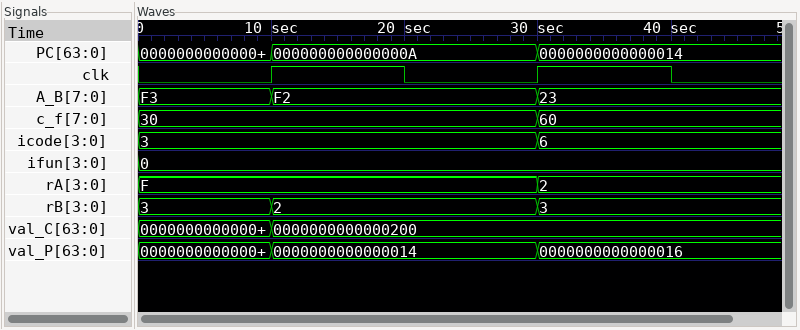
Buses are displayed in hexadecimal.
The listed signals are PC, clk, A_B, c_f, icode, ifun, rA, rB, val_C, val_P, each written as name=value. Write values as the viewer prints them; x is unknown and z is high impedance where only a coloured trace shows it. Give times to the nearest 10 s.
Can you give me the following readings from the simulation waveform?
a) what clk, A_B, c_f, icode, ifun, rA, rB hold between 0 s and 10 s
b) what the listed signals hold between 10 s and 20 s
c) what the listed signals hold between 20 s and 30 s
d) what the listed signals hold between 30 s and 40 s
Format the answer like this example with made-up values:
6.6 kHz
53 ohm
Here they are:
clk=0, A_B=F3, c_f=30, icode=3, ifun=0, rA=F, rB=3
PC=000000000000000A, clk=1, A_B=F2, c_f=30, icode=3, ifun=0, rA=F, rB=2, val_C=0000000000000200, val_P=0000000000000014
PC=000000000000000A, clk=0, A_B=F2, c_f=30, icode=3, ifun=0, rA=F, rB=2, val_C=0000000000000200, val_P=0000000000000014
PC=0000000000000014, clk=1, A_B=23, c_f=60, icode=6, ifun=0, rA=2, rB=3, val_C=0000000000000200, val_P=0000000000000016
